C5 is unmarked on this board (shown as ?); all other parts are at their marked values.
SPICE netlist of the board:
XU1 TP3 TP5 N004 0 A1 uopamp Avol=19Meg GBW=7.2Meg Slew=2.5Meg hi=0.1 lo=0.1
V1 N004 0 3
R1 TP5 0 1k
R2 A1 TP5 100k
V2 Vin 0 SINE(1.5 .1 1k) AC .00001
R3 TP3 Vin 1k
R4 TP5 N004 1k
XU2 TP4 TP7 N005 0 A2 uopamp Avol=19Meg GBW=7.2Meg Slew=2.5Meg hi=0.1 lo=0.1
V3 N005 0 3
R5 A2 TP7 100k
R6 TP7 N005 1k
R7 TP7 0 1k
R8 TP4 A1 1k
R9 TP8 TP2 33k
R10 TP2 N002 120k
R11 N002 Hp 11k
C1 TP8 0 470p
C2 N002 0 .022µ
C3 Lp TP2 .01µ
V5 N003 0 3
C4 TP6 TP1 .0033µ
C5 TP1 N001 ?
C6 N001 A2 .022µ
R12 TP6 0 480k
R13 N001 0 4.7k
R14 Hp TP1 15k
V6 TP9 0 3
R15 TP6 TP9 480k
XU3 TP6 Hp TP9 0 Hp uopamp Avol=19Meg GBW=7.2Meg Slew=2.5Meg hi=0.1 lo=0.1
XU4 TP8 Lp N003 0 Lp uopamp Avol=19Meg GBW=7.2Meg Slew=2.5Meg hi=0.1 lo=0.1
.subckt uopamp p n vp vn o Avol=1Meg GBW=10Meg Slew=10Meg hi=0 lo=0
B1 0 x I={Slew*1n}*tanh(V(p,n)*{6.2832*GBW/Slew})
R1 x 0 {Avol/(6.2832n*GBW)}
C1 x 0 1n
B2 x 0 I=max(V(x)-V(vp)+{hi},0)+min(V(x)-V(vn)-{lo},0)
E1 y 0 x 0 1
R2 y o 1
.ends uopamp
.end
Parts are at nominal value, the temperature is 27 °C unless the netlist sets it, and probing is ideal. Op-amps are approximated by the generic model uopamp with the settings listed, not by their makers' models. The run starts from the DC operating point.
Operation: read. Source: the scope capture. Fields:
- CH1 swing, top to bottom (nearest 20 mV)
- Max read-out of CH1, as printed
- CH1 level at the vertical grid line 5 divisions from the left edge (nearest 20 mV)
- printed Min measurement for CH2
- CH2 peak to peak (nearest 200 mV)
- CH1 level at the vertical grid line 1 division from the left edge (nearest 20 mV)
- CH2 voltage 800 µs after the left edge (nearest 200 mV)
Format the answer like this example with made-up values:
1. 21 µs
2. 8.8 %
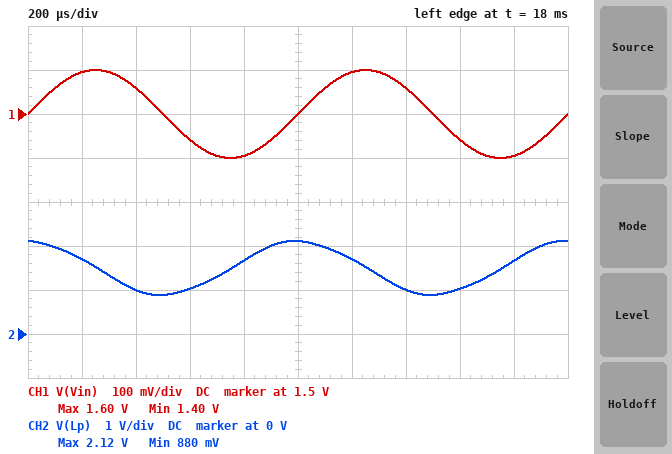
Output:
1. 200 mV
2. 1.60 V
3. 1.50 V
4. 880 mV
5. 1.2 V
6. 1.60 V
7. 1.6 V
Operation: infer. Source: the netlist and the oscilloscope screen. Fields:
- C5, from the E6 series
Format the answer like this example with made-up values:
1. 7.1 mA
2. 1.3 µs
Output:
1. 1 nF
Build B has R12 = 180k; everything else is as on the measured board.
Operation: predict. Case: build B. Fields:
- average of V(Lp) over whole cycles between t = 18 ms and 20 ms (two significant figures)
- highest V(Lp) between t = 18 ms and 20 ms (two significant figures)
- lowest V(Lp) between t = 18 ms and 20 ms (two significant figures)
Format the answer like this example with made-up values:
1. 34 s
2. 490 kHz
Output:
1. 830 mV
2. 1.1 V
3. 570 mV
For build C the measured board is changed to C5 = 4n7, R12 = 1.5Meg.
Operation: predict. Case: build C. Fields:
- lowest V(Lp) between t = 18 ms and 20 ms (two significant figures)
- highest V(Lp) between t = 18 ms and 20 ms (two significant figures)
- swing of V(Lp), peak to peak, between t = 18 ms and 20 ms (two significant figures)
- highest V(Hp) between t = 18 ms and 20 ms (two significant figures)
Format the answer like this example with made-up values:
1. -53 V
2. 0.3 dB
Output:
1. 1.4 V
2. 2.9 V
3. 1.5 V
4. 2.9 V
